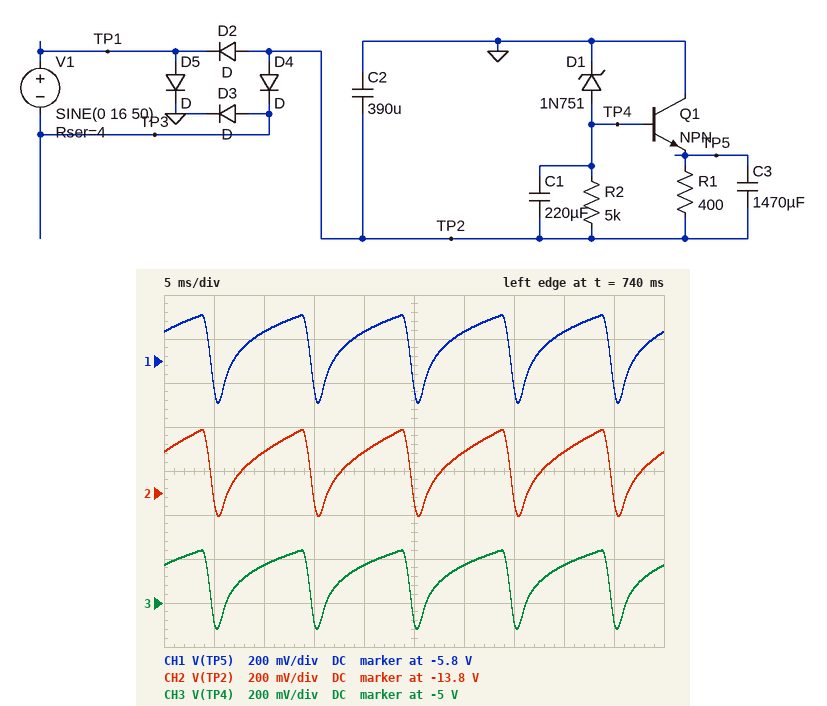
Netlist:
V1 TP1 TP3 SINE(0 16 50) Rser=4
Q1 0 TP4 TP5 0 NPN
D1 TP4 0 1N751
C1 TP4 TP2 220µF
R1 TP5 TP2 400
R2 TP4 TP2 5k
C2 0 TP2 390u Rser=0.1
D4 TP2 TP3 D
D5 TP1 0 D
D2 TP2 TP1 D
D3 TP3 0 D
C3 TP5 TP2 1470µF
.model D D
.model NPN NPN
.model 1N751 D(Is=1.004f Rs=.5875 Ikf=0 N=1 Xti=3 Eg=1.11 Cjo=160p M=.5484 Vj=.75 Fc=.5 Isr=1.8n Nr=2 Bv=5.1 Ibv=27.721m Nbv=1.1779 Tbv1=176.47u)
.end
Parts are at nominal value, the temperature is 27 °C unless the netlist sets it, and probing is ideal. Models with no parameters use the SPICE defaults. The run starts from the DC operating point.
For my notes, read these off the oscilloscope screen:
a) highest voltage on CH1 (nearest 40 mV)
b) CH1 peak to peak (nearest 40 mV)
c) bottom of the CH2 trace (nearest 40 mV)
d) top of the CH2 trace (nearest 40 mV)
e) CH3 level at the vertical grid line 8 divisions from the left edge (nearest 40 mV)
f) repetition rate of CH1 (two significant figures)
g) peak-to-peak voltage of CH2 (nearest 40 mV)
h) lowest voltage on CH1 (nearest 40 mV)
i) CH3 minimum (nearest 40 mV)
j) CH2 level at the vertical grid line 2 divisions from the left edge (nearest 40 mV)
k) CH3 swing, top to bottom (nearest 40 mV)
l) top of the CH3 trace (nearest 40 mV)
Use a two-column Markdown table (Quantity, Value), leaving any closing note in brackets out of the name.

| Quantity | Value |
|---|---|
| highest voltage on CH1 | -5.60 V |
| CH1 peak to peak | 400 mV |
| bottom of the CH2 trace | -13.92 V |
| top of the CH2 trace | -13.52 V |
| CH3 level at the vertical grid line 8 divisions from the left edge | -4.84 V |
| repetition rate of CH1 | 100 Hz |
| peak-to-peak voltage of CH2 | 400 mV |
| lowest voltage on CH1 | -6.00 V |
| CH3 minimum | -5.12 V |
| CH2 level at the vertical grid line 2 divisions from the left edge | -13.60 V |
| CH3 swing, top to bottom | 360 mV |
| top of the CH3 trace | -4.76 V |
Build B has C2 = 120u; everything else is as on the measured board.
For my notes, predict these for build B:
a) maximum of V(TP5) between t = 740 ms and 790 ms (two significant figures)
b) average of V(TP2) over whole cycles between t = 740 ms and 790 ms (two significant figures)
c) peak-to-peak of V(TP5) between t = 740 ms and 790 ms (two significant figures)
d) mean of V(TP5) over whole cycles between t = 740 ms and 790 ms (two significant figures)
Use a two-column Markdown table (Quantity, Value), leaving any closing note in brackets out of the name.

| Quantity | Value |
|---|---|
| maximum of V(TP5) between t = 740 ms and 790 ms | -4.9 V |
| average of V(TP2) over whole cycles between t = 740 ms and 790 ms | -13 V |
| peak-to-peak of V(TP5) between t = 740 ms and 790 ms | 1.1 V |
| mean of V(TP5) over whole cycles between t = 740 ms and 790 ms | -5.3 V |
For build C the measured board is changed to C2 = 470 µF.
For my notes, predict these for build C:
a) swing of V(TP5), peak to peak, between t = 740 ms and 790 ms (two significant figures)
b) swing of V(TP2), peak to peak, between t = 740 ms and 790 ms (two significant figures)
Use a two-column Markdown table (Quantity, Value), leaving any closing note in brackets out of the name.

| Quantity | Value |
|---|---|
| swing of V(TP5), peak to peak, between t = 740 ms and 790 ms | 340 mV |
| swing of V(TP2), peak to peak, between t = 740 ms and 790 ms | 330 mV |
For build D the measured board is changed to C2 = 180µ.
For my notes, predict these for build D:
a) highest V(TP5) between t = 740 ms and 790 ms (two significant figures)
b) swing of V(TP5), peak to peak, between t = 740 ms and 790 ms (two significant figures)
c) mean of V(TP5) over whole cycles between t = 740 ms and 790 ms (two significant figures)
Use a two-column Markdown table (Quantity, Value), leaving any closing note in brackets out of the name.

| Quantity | Value |
|---|---|
| highest V(TP5) between t = 740 ms and 790 ms | -5.2 V |
| swing of V(TP5), peak to peak, between t = 740 ms and 790 ms | 800 mV |
| mean of V(TP5) over whole cycles between t = 740 ms and 790 ms | -5.5 V |
